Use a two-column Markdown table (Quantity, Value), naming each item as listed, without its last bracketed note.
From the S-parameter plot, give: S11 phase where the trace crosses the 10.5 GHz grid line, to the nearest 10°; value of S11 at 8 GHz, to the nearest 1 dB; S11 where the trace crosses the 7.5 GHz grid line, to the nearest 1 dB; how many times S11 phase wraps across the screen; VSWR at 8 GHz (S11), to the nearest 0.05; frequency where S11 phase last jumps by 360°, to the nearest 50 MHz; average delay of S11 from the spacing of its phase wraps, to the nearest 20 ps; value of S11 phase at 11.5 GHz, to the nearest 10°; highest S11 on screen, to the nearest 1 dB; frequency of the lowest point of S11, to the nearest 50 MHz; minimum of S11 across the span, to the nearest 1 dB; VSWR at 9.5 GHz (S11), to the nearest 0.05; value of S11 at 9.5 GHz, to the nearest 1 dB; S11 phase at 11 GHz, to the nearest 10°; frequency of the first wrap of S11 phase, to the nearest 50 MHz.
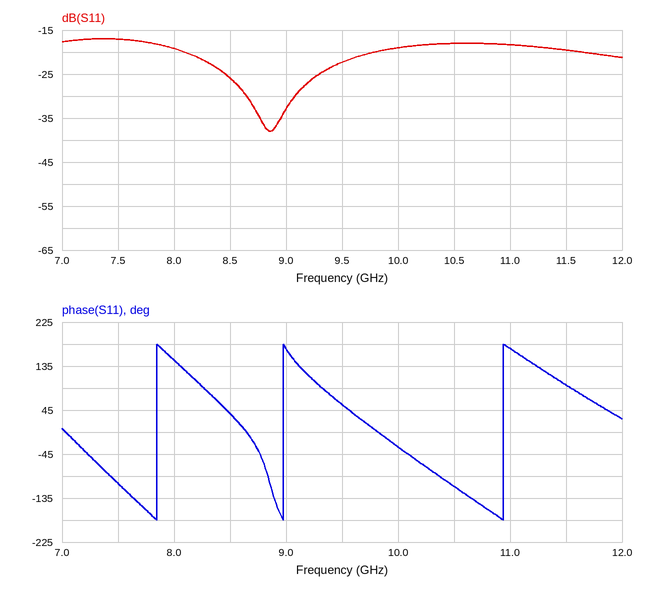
| Quantity | Value |
|---|---|
| S11 phase where the trace crosses the 10.5 GHz grid line, to the nearest 10° | -110° |
| value of S11 at 8 GHz, to the nearest 1 dB | -19 dB |
| S11 where the trace crosses the 7.5 GHz grid line, to the nearest 1 dB | -17 dB |
| how many times S11 phase wraps across the screen | 3 |
| VSWR at 8 GHz (S11), to the nearest 0.05 | 1.25 |
| frequency where S11 phase last jumps by 360°, to the nearest 50 MHz | 10.95 GHz |
| average delay of S11 from the spacing of its phase wraps, to the nearest 20 ps | 640 ps |
| value of S11 phase at 11.5 GHz, to the nearest 10° | 100° |
| highest S11 on screen, to the nearest 1 dB | -17 dB |
| frequency of the lowest point of S11, to the nearest 50 MHz | 8.85 GHz |
| minimum of S11 across the span, to the nearest 1 dB | -38 dB |
| VSWR at 9.5 GHz (S11), to the nearest 0.05 | 1.15 |
| value of S11 at 9.5 GHz, to the nearest 1 dB | -22 dB |
| S11 phase at 11 GHz, to the nearest 10° | 170° |
| frequency of the first wrap of S11 phase, to the nearest 50 MHz | 7.85 GHz |
